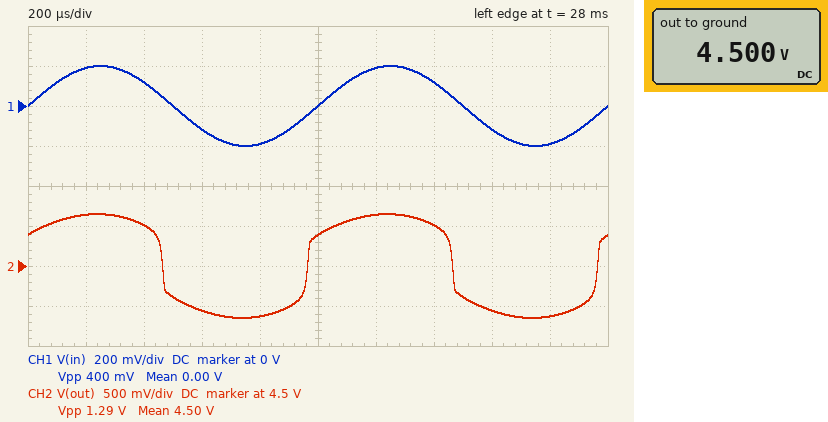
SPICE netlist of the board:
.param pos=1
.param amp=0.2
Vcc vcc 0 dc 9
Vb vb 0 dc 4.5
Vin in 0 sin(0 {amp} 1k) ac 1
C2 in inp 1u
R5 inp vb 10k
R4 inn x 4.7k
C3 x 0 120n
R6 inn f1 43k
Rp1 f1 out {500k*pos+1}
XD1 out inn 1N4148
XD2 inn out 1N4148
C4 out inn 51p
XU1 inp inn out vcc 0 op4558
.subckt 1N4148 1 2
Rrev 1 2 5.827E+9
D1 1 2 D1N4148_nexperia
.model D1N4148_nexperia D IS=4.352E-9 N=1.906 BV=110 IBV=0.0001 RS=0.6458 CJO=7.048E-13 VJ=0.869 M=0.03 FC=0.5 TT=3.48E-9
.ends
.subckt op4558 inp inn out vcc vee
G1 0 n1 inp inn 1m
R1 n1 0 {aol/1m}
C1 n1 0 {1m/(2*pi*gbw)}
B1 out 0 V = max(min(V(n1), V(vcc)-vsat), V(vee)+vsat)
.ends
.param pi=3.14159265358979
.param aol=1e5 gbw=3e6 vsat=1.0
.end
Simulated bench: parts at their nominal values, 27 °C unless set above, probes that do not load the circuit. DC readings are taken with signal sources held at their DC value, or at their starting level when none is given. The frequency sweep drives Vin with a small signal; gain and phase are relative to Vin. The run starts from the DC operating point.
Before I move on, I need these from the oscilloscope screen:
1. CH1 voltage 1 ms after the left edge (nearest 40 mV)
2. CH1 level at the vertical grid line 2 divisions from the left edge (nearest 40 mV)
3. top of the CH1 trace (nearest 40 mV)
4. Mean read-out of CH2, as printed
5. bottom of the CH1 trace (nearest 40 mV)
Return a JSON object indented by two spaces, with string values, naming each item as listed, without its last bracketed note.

{
  "CH1 voltage 1 ms after the left edge": "0 V",
  "CH1 level at the vertical grid line 2 divisions from the left edge": "120 mV",
  "top of the CH1 trace": "200 mV",
  "Mean read-out of CH2, as printed": "4.50 V",
  "bottom of the CH1 trace": "-200 mV"
}
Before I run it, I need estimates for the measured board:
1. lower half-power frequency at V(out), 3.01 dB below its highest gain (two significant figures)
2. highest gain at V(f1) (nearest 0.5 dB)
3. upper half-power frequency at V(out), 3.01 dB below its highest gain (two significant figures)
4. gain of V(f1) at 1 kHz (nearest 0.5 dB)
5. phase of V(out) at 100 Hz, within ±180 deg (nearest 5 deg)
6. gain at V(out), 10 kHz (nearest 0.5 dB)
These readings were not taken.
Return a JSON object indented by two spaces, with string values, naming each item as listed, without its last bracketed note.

{
  "lower half-power frequency at V(out), 3.01 dB below its highest gain": "260 Hz",
  "highest gain at V(f1)": "19.0 dB",
  "upper half-power frequency at V(out), 3.01 dB below its highest gain": "5.5 kHz",
  "gain of V(f1) at 1 kHz": "19.0 dB",
  "phase of V(out) at 100 Hz, within ±180 deg": "75 deg",
  "gain at V(out), 10 kHz": "33.5 dB"
}
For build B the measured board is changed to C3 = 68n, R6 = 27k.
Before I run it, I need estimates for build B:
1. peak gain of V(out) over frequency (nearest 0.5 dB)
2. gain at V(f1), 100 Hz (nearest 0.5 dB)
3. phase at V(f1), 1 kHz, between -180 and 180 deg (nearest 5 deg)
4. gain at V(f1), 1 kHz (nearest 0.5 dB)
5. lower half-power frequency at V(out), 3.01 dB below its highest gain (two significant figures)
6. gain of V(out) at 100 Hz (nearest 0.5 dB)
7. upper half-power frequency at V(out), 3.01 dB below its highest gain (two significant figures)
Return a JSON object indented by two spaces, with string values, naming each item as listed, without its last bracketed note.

{
  "peak gain of V(out) over frequency": "39.5 dB",
  "gain at V(f1), 100 Hz": "4.0 dB",
  "phase at V(f1), 1 kHz, between -180 and 180 deg": "15 deg",
  "gain at V(f1), 1 kHz": "15.0 dB",
  "lower half-power frequency at V(out), 3.01 dB below its highest gain": "430 Hz",
  "gain of V(out) at 100 Hz": "26.0 dB",
  "upper half-power frequency at V(out), 3.01 dB below its highest gain": "6.0 kHz"
}
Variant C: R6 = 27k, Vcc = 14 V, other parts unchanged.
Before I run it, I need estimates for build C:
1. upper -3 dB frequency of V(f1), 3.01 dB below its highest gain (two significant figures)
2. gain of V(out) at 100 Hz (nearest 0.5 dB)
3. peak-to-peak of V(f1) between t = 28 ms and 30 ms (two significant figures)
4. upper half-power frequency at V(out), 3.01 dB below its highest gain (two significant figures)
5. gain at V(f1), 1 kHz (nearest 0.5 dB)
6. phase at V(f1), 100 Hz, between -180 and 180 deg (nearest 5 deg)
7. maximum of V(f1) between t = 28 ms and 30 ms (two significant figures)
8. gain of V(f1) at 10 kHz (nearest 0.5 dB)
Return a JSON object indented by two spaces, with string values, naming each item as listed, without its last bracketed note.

{
  "upper -3 dB frequency of V(f1), 3.01 dB below its highest gain": "5.8 kHz",
  "gain of V(out) at 100 Hz": "30.5 dB",
  "peak-to-peak of V(f1) between t = 28 ms and 30 ms": "450 mV",
  "upper half-power frequency at V(out), 3.01 dB below its highest gain": "5.7 kHz",
  "gain at V(f1), 1 kHz": "15.5 dB",
  "phase at V(f1), 100 Hz, between -180 and 180 deg": "55 deg",
  "maximum of V(f1) between t = 28 ms and 30 ms": "4.7 V",
  "gain of V(f1) at 10 kHz": "9.5 dB"
}
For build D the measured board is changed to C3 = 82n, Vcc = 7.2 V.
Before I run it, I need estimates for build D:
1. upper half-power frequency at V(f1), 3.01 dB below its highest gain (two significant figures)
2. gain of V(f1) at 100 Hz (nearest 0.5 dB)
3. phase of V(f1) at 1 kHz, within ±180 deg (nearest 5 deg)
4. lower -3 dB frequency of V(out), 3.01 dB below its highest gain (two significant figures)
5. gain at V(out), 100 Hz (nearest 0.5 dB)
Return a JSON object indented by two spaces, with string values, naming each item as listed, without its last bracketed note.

{
  "upper half-power frequency at V(f1), 3.01 dB below its highest gain": "5.8 kHz",
  "gain of V(f1) at 100 Hz": "7.5 dB",
  "phase of V(f1) at 1 kHz, within ±180 deg": "10 deg",
  "lower -3 dB frequency of V(out), 3.01 dB below its highest gain": "360 Hz",
  "gain at V(out), 100 Hz": "28.0 dB"
}
